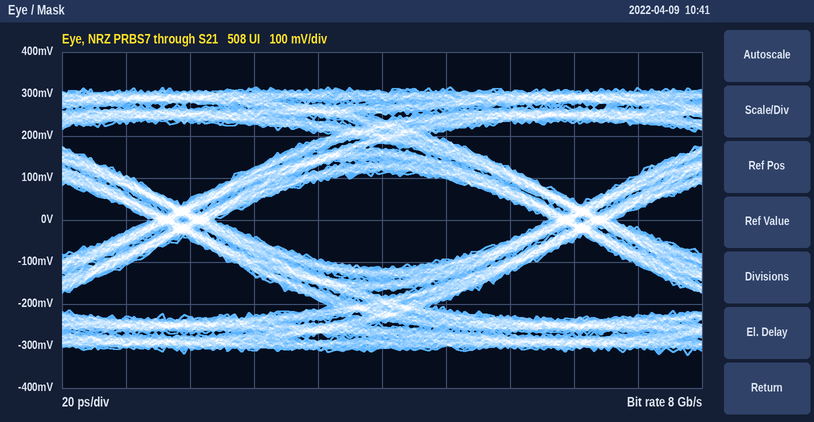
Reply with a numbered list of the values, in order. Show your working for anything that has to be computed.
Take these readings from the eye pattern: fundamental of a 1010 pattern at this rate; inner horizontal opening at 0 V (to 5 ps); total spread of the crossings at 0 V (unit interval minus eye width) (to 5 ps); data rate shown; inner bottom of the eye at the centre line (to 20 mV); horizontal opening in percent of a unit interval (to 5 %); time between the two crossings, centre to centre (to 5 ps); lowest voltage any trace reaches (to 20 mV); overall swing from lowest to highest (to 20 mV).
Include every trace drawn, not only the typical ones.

1. 4 GHz
2. 105 ps
3. 20 ps
4. 8 Gb/s
5. -120 mV
6. 105 ps / 125 ps ≈ 84.0 %, so 85 % to the nearest 5 %
7. 125 ps
8. -320 mV
9. 640 mV
